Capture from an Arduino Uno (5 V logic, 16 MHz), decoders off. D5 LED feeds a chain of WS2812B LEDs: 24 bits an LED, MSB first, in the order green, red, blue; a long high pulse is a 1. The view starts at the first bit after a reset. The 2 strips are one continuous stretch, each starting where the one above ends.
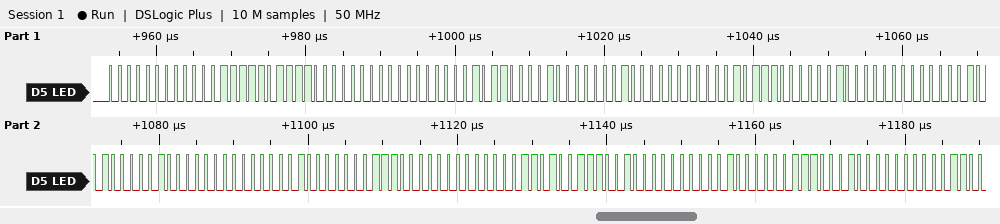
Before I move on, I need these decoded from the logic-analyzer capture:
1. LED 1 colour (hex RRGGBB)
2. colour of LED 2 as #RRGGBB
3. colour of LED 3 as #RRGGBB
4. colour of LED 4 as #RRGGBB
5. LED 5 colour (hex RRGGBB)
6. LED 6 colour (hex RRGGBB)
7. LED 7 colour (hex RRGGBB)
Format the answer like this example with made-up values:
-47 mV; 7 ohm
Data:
#0F00BC; #010061; #000117; #000209; #000408; #000E0D; #003920
